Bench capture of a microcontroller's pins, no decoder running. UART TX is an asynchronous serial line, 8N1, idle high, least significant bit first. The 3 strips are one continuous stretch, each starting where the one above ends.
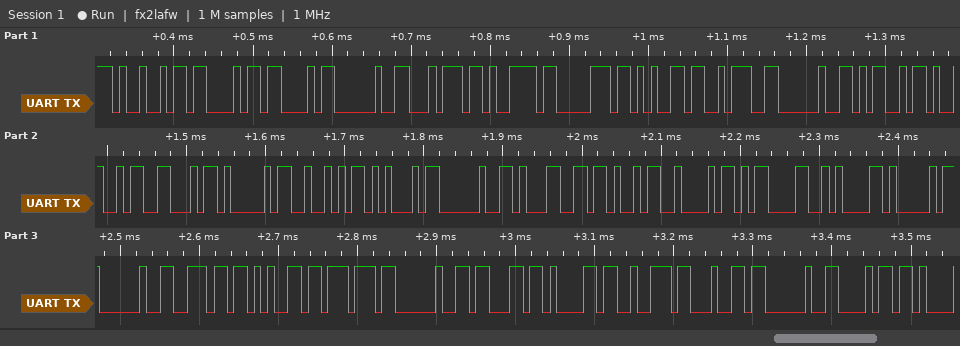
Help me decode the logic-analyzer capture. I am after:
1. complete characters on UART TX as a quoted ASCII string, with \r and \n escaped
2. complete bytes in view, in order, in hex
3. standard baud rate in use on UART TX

"ICC type: MIFARE 1KB\r\nA new card h"
0x49 0x43 0x43 0x20 0x74 0x79 0x70 0x65 0x3A 0x20 0x4D 0x49 0x46 0x41 0x52 0x45 0x20 0x31 0x4B 0x42 0x0D 0x0A 0x41 0x20 0x6E 0x65 0x77 0x20 0x63 0x61 0x72 0x64 0x20 0x68
115200 baud
